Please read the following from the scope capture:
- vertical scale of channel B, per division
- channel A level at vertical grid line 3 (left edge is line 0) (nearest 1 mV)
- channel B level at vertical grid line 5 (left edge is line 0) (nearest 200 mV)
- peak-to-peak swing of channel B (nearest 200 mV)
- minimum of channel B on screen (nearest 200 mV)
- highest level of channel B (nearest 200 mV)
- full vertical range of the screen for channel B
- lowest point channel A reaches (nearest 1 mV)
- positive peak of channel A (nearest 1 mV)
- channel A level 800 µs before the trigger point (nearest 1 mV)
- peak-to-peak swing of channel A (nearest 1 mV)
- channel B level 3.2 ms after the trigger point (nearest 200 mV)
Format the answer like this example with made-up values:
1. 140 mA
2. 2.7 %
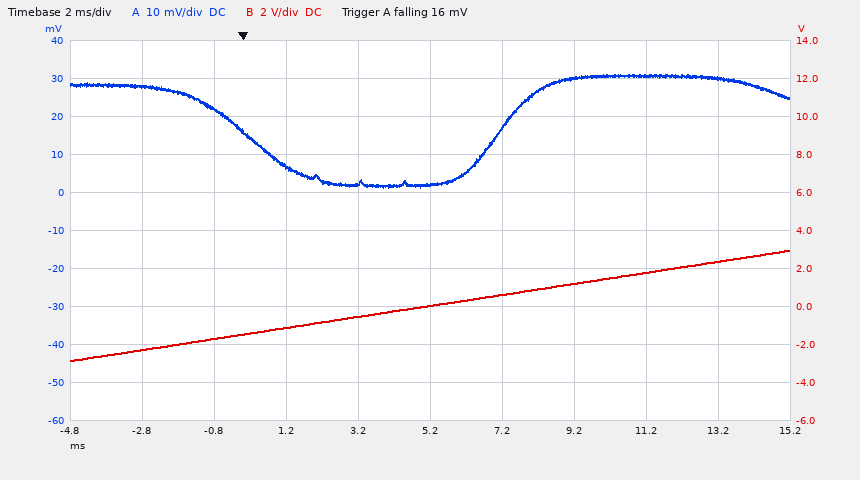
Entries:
1. 2 V
2. 7 mV
3. 0.0 V
4. 5.8 V
5. -2.8 V
6. 3.0 V
7. 20 V
8. 1 mV
9. 31 mV
10. 22 mV
11. 30 mV
12. -600 mV
